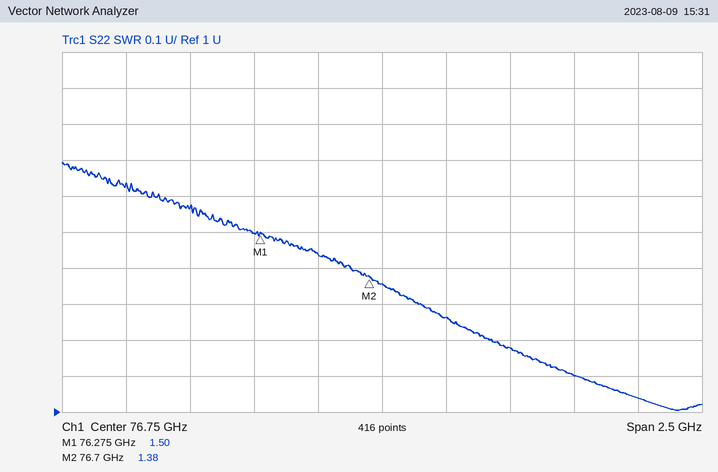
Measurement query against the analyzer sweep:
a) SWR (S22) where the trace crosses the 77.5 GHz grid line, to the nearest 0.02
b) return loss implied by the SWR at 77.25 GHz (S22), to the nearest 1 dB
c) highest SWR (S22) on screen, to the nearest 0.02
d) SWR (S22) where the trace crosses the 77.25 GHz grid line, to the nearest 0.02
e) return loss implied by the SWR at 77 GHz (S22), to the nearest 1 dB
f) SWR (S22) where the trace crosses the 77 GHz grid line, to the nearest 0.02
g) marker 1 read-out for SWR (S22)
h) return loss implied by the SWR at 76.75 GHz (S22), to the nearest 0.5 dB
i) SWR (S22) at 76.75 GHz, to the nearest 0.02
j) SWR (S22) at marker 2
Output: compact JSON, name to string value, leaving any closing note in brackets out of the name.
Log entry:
{"SWR (S22) where the trace crosses the 77.5 GHz grid line, to the nearest 0.02": "1.10", "return loss implied by the SWR at 77.25 GHz (S22), to the nearest 1 dB": "22 dB", "highest SWR (S22) on screen, to the nearest 0.02": "1.70", "SWR (S22) where the trace crosses the 77.25 GHz grid line, to the nearest 0.02": "1.18", "return loss implied by the SWR at 77 GHz (S22), to the nearest 1 dB": "19 dB", "SWR (S22) where the trace crosses the 77 GHz grid line, to the nearest 0.02": "1.26", "marker 1 read-out for SWR": "1.50", "return loss implied by the SWR at 76.75 GHz (S22), to the nearest 0.5 dB": "16.5 dB", "SWR (S22) at 76.75 GHz, to the nearest 0.02": "1.36", "SWR (S22) at marker 2": "1.38"}
